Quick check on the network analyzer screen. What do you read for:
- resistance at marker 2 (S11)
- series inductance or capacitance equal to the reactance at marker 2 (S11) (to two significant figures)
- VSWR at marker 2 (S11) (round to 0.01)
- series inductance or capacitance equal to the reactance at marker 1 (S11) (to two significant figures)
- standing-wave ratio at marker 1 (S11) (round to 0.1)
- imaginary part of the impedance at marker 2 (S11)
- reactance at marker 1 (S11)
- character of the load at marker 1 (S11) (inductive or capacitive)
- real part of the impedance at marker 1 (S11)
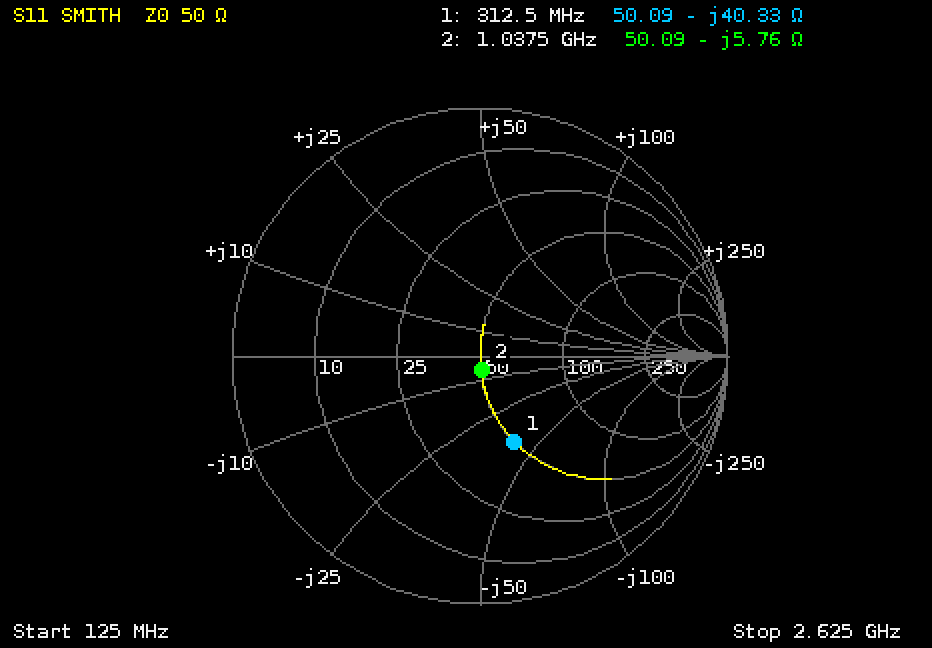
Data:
50.09 Ω
27 pF
1.12
13 pF
2.2
-5.76 Ω
-40.33 Ω
capacitive
50.09 Ω
